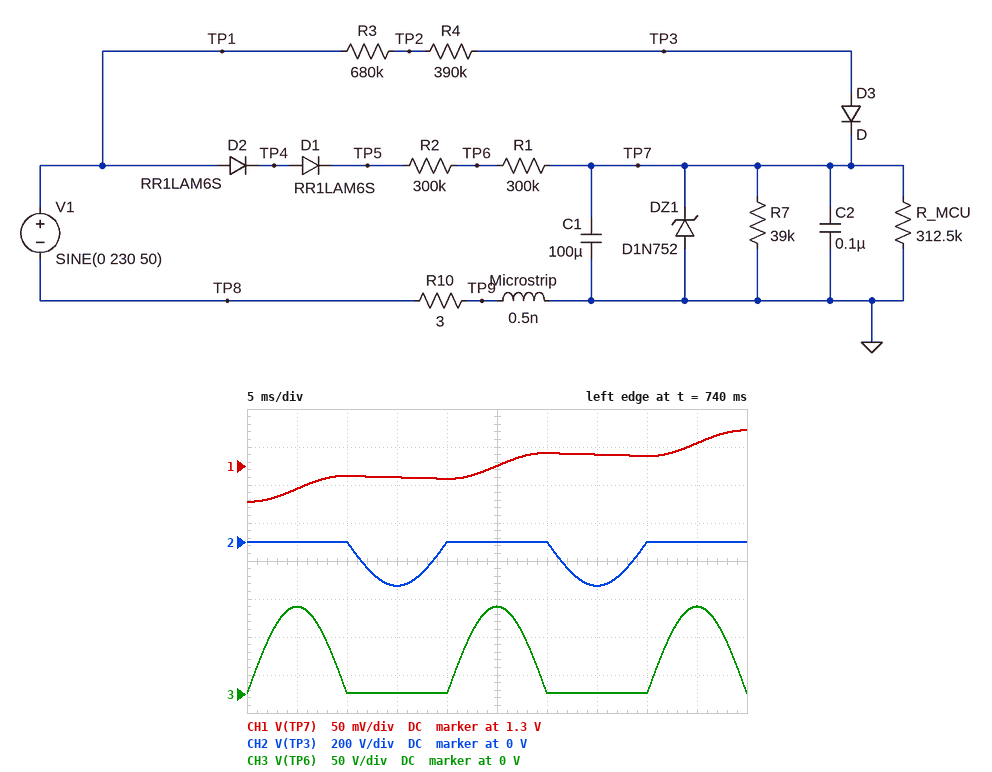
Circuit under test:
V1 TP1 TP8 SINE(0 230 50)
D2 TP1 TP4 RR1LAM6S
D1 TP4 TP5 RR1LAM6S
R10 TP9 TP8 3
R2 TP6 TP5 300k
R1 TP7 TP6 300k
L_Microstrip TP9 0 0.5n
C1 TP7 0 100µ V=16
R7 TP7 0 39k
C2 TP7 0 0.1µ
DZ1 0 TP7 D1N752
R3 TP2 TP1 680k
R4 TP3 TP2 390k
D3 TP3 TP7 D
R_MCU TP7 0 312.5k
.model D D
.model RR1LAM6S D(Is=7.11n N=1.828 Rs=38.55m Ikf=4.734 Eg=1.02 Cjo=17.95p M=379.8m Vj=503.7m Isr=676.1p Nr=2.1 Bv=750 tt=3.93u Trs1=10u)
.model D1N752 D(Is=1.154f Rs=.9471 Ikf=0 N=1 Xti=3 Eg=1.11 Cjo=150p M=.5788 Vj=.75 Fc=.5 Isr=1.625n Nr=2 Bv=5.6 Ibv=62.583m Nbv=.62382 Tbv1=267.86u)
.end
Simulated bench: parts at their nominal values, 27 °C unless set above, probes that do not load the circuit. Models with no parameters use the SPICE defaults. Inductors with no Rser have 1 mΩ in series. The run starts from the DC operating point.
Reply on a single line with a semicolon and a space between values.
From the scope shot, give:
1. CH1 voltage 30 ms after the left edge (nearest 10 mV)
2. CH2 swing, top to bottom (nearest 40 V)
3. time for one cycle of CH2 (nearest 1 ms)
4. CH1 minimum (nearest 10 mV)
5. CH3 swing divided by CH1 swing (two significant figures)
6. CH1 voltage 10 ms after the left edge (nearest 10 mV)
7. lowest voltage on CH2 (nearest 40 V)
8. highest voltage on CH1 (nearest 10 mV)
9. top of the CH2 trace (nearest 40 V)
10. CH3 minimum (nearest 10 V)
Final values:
1.32 V; 240 V; 20 ms; 1.25 V; 1200; 1.29 V; -240 V; 1.35 V; 0 V; 0 V
